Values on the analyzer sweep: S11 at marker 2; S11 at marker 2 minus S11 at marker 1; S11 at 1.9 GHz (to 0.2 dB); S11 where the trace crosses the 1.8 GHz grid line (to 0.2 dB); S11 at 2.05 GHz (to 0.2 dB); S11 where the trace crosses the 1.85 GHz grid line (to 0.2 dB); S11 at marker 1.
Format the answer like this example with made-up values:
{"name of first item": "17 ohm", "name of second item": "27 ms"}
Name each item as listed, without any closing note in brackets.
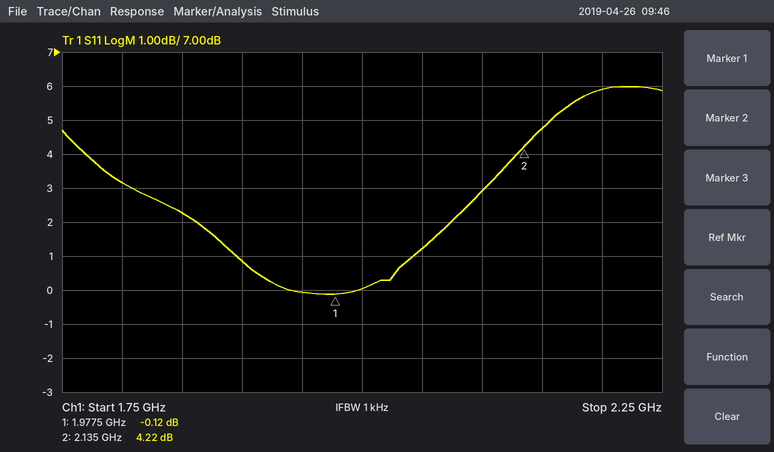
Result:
{"S11 at marker 2": "4.22 dB", "S11 at marker 2 minus S11 at marker 1": "4.34 dB", "S11 at 1.9 GHz": "0.8 dB", "S11 where the trace crosses the 1.8 GHz grid line": "3.2 dB", "S11 at 2.05 GHz": "1.2 dB", "S11 where the trace crosses the 1.85 GHz grid line": "2.2 dB", "S11 at marker 1": "-0.12 dB"}
